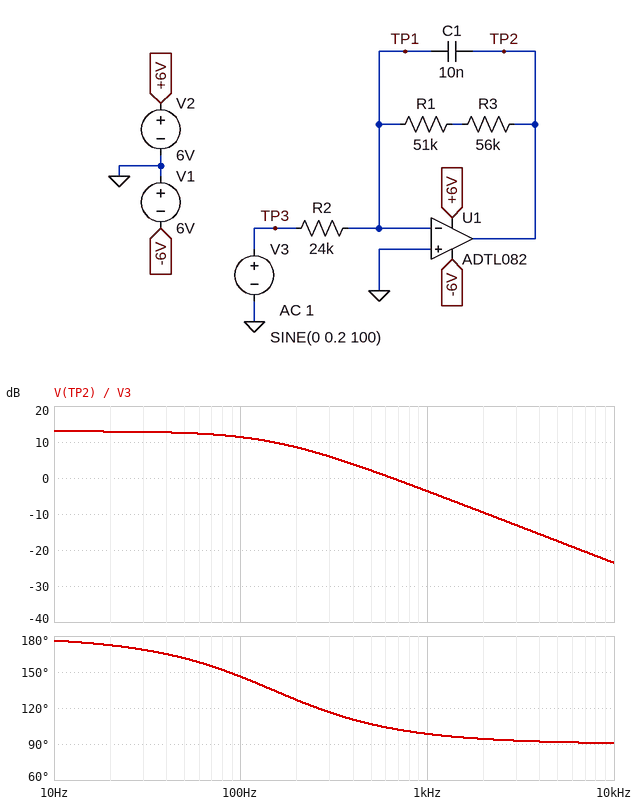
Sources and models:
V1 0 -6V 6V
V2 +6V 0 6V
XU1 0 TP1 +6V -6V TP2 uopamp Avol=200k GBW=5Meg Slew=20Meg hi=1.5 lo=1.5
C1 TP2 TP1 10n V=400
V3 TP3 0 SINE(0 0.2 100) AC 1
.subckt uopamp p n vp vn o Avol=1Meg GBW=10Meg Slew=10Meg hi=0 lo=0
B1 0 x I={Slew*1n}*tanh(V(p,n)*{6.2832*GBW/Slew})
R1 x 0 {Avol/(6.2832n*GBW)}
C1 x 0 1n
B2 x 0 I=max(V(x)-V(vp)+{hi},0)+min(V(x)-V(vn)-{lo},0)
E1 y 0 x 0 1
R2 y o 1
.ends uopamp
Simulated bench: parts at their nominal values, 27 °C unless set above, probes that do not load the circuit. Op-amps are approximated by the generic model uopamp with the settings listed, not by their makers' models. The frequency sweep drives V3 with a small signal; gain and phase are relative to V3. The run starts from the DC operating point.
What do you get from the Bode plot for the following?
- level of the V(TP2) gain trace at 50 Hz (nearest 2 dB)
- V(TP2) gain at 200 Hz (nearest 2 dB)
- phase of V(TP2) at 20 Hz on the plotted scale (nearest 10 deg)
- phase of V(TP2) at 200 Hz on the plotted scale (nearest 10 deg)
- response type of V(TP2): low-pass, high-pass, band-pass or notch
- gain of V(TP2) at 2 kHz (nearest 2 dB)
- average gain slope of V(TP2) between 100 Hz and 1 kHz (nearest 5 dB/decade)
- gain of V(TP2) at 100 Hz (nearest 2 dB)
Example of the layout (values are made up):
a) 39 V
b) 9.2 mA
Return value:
a) 12 dB
b) 8 dB
c) 170 deg
d) 130 deg
e) low-pass
f) -10 dB
g) -15 dB/decade
h) 12 dB
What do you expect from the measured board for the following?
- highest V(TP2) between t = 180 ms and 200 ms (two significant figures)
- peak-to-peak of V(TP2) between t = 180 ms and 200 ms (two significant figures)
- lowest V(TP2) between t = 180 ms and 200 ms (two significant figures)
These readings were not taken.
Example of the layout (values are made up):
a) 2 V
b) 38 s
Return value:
a) 740 mV
b) 1.5 V
c) -740 mV
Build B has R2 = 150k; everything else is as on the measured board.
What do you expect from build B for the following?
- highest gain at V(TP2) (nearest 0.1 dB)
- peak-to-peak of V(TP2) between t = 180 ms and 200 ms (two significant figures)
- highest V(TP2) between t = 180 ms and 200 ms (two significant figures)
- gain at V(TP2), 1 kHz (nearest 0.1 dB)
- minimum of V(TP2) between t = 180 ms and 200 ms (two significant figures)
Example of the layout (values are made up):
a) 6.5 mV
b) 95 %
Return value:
a) -2.9 dB
b) 240 mV
c) 120 mV
d) -19.6 dB
e) -120 mV
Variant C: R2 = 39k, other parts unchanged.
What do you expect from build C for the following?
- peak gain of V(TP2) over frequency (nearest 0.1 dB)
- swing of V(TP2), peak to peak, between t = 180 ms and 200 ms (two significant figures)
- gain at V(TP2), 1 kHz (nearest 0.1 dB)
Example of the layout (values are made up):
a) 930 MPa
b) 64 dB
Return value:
a) 8.8 dB
b) 910 mV
c) -7.9 dB
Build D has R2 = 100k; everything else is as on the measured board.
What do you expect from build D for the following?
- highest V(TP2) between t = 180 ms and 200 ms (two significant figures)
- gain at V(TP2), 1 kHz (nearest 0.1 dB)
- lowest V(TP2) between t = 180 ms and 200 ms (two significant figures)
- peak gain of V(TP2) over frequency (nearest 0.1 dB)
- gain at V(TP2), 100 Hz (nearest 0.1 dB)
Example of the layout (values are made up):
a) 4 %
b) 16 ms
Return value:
a) 180 mV
b) -16.1 dB
c) -180 mV
d) 0.6 dB
e) -1.0 dB
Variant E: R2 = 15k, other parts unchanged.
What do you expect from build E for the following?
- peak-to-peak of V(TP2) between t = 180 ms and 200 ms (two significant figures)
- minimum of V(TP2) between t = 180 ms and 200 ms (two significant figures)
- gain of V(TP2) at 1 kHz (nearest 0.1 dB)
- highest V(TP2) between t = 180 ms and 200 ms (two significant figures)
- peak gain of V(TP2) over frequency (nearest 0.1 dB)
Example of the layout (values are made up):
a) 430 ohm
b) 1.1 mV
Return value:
a) 2.4 V
b) -1.2 V
c) 0.4 dB
d) 1.2 V
e) 17.1 dB
